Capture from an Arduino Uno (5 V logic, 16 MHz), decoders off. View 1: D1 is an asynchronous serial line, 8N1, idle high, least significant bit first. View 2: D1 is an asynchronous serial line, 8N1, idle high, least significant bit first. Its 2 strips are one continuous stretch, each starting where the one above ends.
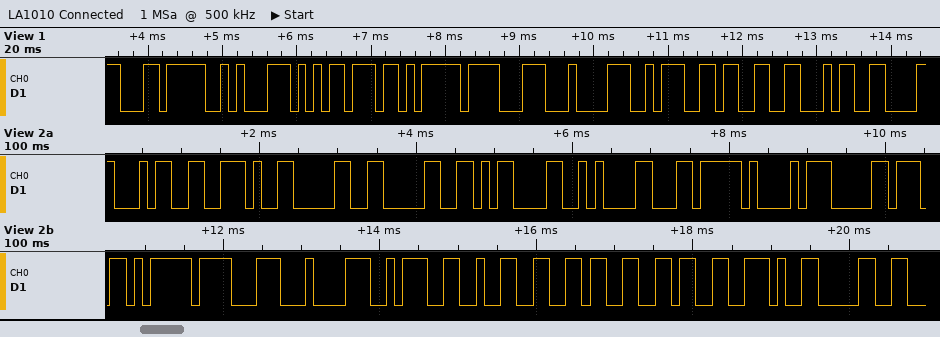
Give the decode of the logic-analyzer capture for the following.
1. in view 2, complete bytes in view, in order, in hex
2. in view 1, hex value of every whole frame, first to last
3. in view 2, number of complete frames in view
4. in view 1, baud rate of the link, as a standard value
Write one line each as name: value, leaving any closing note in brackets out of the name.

in view 2, complete bytes in view, in order, in hex: 34 2E 30 30 0D 0A EC A1 B0 EB 8F 84 3A 32 36 36 2E 30
in view 1, hex value of every whole frame, first to last: EC 8A B5 EB 8F 84 3A 33 34
in view 2, number of complete frames in view: 18
in view 1, baud rate of the link, as a standard value: 9600 baud
